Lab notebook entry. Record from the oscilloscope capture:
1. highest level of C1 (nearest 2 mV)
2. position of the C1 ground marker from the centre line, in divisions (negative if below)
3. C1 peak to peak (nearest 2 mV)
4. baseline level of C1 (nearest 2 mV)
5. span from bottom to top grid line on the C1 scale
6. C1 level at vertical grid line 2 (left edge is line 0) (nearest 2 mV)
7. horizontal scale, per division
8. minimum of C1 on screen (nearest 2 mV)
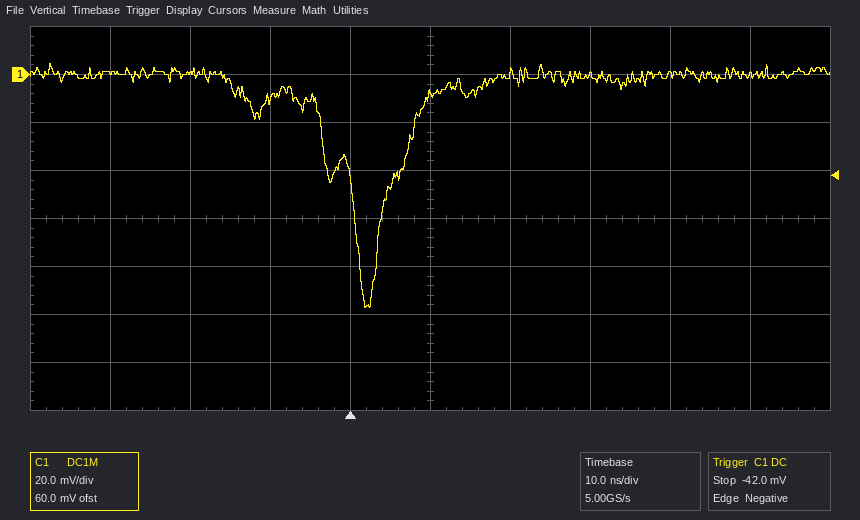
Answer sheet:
4 mV
+3.0 div
102 mV
0 mV
160 mV
2 mV
10 ns
-98 mV
